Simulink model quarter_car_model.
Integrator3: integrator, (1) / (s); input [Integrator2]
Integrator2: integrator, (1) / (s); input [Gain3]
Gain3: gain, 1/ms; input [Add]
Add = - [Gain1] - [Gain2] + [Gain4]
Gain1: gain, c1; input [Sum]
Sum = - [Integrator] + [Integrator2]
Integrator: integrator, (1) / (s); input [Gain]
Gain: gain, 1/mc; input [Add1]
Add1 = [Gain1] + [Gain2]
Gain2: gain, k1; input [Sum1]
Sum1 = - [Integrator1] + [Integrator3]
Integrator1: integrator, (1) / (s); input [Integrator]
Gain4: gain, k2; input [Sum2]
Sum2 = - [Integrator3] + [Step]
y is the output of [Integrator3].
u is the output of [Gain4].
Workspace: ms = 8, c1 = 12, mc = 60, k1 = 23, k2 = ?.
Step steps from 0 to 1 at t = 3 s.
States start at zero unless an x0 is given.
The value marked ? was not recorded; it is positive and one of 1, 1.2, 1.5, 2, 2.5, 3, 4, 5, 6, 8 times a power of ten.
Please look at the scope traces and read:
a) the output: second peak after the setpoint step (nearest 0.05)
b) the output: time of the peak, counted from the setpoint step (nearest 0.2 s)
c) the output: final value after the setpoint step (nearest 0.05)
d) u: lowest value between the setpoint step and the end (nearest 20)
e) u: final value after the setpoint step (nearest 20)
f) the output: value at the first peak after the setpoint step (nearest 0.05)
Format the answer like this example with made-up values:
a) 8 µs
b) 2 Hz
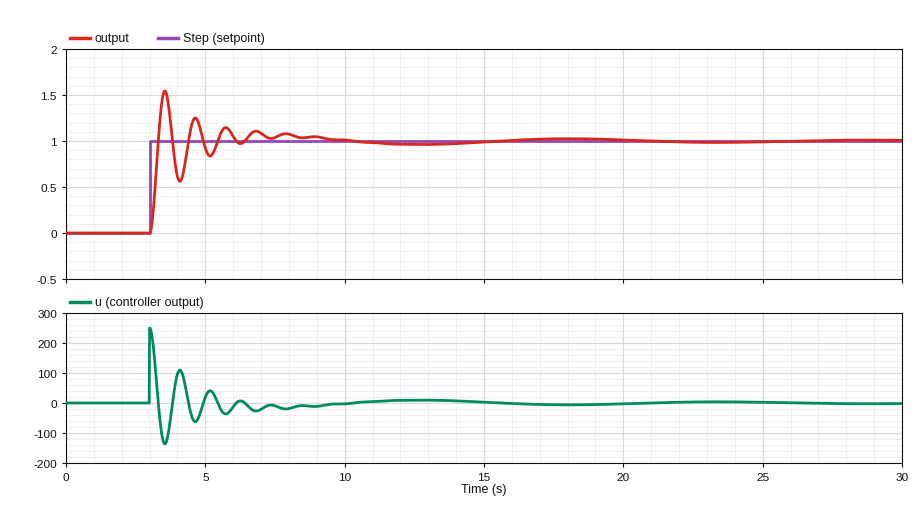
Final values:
a) 1.25
b) 0.6 s
c) 1.00
d) -140
e) 0
f) 1.55
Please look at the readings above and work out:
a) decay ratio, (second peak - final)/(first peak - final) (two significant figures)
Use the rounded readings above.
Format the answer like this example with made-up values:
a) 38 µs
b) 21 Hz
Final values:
a) 0.45
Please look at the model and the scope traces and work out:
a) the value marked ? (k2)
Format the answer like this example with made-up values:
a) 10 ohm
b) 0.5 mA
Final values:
a) 250
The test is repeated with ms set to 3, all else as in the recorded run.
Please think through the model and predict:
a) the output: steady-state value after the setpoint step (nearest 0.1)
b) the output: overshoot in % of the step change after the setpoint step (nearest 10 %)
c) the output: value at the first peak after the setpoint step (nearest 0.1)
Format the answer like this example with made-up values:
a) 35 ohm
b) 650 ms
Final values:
a) 1.0
b) 40 %
c) 1.4
